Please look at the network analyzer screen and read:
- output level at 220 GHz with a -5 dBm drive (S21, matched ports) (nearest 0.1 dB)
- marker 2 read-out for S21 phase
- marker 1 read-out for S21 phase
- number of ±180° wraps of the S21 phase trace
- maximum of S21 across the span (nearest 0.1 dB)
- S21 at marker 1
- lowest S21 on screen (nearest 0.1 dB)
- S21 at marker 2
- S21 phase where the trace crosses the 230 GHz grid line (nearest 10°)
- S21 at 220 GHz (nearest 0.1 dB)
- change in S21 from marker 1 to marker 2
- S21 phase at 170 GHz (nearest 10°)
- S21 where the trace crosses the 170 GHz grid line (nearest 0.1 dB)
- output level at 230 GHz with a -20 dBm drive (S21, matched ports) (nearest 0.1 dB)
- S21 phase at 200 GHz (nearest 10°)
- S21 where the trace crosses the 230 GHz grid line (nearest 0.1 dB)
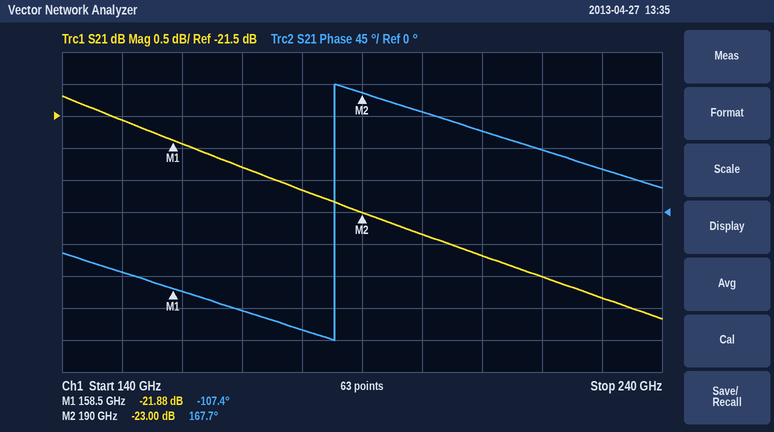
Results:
-29.0 dBm
167.7°
-107.4°
1
-21.2 dB
-21.88 dB
-24.7 dB
-23.00 dB
60°
-24.0 dB
-1.12 dB
-140°
-22.3 dB
-44.3 dBm
140°
-24.3 dB
